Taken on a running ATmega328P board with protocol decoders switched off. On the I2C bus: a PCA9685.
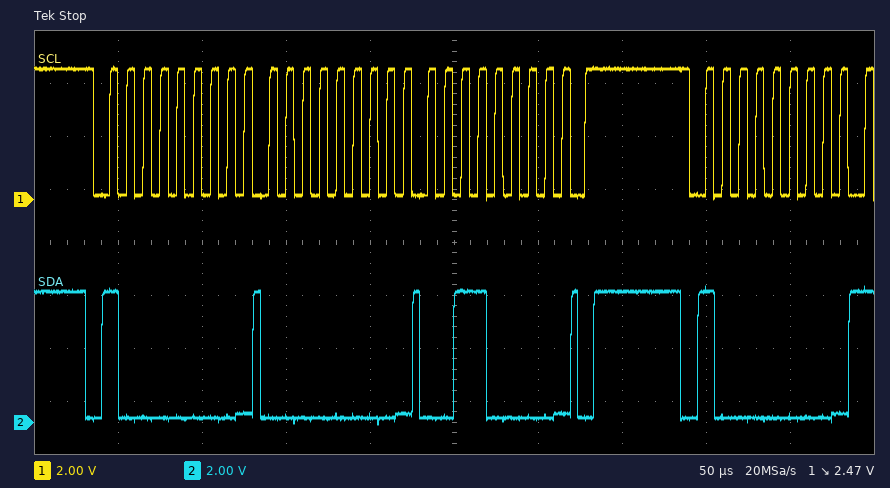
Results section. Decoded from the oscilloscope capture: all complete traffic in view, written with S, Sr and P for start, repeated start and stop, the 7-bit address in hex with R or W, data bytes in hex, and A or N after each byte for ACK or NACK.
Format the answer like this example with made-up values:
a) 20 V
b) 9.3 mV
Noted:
a) S 40W A 00 A 30 A P S 40W A
